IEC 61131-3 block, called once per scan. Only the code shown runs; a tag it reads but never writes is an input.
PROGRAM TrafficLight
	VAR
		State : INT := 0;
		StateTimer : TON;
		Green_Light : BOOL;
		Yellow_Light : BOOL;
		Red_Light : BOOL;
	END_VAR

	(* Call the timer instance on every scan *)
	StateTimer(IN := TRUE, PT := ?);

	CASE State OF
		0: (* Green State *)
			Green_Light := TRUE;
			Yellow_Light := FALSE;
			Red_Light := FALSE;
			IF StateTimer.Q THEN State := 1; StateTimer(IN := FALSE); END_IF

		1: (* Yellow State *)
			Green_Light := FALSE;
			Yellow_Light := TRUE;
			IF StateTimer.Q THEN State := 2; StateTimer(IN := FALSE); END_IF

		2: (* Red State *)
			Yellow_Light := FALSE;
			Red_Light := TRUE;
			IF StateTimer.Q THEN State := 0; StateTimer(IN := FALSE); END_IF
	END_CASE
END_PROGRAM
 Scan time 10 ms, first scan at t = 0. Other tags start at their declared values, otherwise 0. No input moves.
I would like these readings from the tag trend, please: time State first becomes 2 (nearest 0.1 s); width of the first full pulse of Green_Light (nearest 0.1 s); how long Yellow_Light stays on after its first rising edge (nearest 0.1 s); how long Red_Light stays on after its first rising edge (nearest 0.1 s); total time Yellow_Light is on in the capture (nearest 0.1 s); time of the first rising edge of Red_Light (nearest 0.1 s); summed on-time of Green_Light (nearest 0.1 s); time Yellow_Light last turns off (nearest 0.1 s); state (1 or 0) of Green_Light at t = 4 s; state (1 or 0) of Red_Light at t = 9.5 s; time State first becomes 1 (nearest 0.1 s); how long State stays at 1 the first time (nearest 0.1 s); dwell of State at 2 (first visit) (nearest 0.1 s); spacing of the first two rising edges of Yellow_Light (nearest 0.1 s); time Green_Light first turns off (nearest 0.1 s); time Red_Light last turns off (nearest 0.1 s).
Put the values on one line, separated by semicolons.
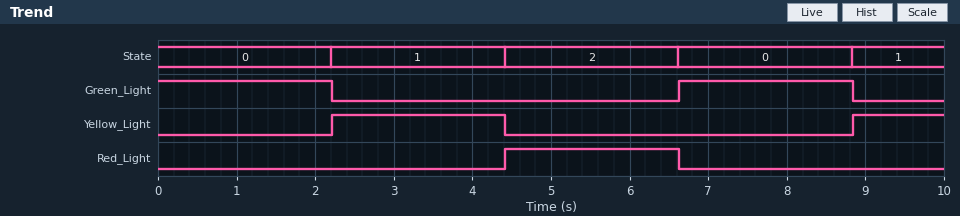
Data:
4.4 s; 2.2 s; 2.2 s; 2.2 s; 3.4 s; 4.4 s; 4.4 s; 4.4 s; 0; 0; 2.2 s; 2.2 s; 2.2 s; 6.6 s; 2.2 s; 6.6 s
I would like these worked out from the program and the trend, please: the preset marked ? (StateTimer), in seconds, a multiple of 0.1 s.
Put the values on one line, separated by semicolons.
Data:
2.2 s
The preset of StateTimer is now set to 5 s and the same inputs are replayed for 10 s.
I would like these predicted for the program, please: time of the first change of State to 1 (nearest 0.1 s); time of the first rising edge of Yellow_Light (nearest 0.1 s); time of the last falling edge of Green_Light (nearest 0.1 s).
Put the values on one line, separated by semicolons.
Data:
5.0 s; 5.0 s; 5.0 s
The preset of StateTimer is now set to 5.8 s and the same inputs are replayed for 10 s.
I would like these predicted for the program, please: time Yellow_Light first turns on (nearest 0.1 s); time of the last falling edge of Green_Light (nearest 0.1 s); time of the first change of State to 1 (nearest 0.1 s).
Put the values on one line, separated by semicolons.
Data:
5.8 s; 5.8 s; 5.8 s
